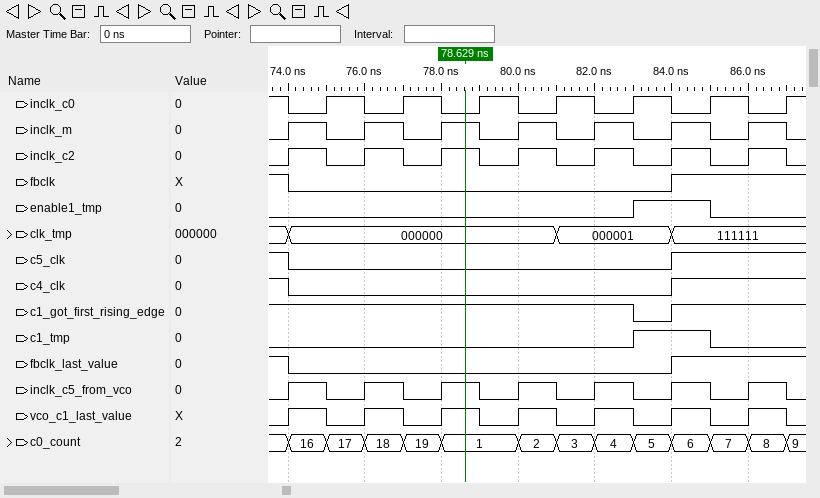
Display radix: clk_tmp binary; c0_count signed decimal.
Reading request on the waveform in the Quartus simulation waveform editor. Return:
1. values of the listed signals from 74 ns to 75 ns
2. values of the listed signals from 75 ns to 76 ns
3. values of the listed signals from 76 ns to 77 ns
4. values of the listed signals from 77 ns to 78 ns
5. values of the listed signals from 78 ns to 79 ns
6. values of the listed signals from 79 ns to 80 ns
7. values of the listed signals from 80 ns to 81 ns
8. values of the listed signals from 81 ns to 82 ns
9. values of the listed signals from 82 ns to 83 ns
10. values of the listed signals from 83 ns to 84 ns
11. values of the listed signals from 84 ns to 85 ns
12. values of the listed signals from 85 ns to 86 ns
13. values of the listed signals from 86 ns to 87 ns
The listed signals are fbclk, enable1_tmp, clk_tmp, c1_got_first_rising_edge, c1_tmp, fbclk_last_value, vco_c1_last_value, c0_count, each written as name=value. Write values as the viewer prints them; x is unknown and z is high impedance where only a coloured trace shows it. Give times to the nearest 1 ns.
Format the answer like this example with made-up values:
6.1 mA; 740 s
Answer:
fbclk=0, enable1_tmp=0, clk_tmp=000000, c1_got_first_rising_edge=1, c1_tmp=0, fbclk_last_value=0, vco_c1_last_value=1, c0_count=16; fbclk=0, enable1_tmp=0, clk_tmp=000000, c1_got_first_rising_edge=1, c1_tmp=0, fbclk_last_value=0, vco_c1_last_value=0, c0_count=17; fbclk=0, enable1_tmp=0, clk_tmp=000000, c1_got_first_rising_edge=1, c1_tmp=0, fbclk_last_value=0, vco_c1_last_value=1, c0_count=18; fbclk=0, enable1_tmp=0, clk_tmp=000000, c1_got_first_rising_edge=1, c1_tmp=0, fbclk_last_value=0, vco_c1_last_value=0, c0_count=19; fbclk=0, enable1_tmp=0, clk_tmp=000000, c1_got_first_rising_edge=1, c1_tmp=0, fbclk_last_value=0, vco_c1_last_value=1, c0_count=1; fbclk=0, enable1_tmp=0, clk_tmp=000000, c1_got_first_rising_edge=1, c1_tmp=0, fbclk_last_value=0, vco_c1_last_value=0, c0_count=1; fbclk=0, enable1_tmp=0, clk_tmp=000000, c1_got_first_rising_edge=1, c1_tmp=0, fbclk_last_value=0, vco_c1_last_value=1, c0_count=2; fbclk=0, enable1_tmp=0, clk_tmp=000001, c1_got_first_rising_edge=1, c1_tmp=0, fbclk_last_value=0, vco_c1_last_value=0, c0_count=3; fbclk=0, enable1_tmp=0, clk_tmp=000001, c1_got_first_rising_edge=1, c1_tmp=0, fbclk_last_value=0, vco_c1_last_value=1, c0_count=4; fbclk=0, enable1_tmp=1, clk_tmp=000001, c1_got_first_rising_edge=0, c1_tmp=1, fbclk_last_value=0, vco_c1_last_value=0, c0_count=5; fbclk=1, enable1_tmp=1, clk_tmp=111111, c1_got_first_rising_edge=1, c1_tmp=1, fbclk_last_value=1, vco_c1_last_value=1, c0_count=6; fbclk=1, enable1_tmp=0, clk_tmp=111111, c1_got_first_rising_edge=1, c1_tmp=0, fbclk_last_value=1, vco_c1_last_value=0, c0_count=7; fbclk=1, enable1_tmp=0, clk_tmp=111111, c1_got_first_rising_edge=1, c1_tmp=0, fbclk_last_value=1, vco_c1_last_value=1, c0_count=8
